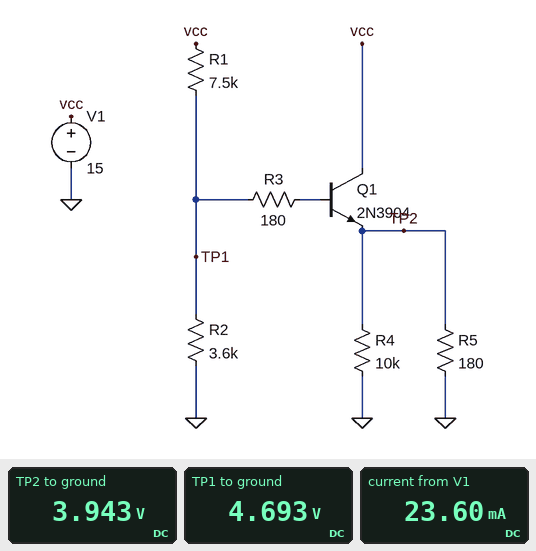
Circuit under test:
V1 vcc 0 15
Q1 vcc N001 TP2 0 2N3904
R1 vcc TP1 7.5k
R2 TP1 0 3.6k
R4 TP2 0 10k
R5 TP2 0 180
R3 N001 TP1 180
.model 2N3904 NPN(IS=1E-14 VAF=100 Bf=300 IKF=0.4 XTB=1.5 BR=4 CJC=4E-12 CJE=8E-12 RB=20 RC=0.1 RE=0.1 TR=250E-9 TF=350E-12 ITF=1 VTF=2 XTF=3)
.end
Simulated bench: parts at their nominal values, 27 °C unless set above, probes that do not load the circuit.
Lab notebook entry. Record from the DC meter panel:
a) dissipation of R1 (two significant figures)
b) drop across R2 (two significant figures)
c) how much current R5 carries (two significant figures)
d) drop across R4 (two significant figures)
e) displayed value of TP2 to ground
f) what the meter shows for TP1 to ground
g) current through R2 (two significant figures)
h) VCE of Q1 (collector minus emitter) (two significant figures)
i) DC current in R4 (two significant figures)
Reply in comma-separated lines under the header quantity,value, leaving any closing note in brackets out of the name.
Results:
quantity,value
dissipation of R1,14 mW
drop across R2,4.7 V
how much current R5 carries,22 mA
drop across R4,3.9 V
displayed value of TP2 to ground,3.943 V
what the meter shows for TP1 to ground,4.693 V
current through R2,1.3 mA
VCE of Q1 (collector minus emitter),11 V
DC current in R4,390 µA
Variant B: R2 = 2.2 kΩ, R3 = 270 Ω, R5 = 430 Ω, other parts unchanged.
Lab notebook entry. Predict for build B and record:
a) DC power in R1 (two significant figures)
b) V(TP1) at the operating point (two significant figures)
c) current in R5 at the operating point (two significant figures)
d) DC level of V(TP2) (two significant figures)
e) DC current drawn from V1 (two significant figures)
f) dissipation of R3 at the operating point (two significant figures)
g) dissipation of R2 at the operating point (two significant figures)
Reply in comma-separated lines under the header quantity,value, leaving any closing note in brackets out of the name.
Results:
quantity,value
DC power in R1,18 mW
V(TP1) at the operating point,3.4 V
current in R5 at the operating point,6.2 mA
DC level of V(TP2),2.7 V
DC current drawn from V1,8.0 mA
dissipation of R3 at the operating point,100 nW
dissipation of R2 at the operating point,5.2 mW
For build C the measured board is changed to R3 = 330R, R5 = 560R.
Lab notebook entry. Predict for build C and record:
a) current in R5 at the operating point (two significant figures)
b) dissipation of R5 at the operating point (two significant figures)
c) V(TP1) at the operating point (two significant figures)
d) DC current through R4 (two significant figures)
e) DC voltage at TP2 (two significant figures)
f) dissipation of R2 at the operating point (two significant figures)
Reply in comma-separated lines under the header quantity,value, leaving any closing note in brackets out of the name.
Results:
quantity,value
current in R5 at the operating point,7.3 mA
dissipation of R5 at the operating point,30 mW
V(TP1) at the operating point,4.8 V
DC current through R4,410 µA
DC voltage at TP2,4.1 V
dissipation of R2 at the operating point,6.4 mW
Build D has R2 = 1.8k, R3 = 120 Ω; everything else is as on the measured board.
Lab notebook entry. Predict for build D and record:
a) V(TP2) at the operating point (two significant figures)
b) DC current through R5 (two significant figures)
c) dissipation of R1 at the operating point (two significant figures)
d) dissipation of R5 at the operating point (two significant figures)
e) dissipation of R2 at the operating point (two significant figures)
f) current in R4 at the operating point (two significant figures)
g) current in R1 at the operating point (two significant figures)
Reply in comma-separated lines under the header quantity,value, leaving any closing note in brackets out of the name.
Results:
quantity,value
V(TP2) at the operating point,2.1 V
DC current through R5,12 mA
dissipation of R1 at the operating point,20 mW
dissipation of R5 at the operating point,25 mW
dissipation of R2 at the operating point,4.5 mW
current in R4 at the operating point,210 µA
current in R1 at the operating point,1.6 mA
